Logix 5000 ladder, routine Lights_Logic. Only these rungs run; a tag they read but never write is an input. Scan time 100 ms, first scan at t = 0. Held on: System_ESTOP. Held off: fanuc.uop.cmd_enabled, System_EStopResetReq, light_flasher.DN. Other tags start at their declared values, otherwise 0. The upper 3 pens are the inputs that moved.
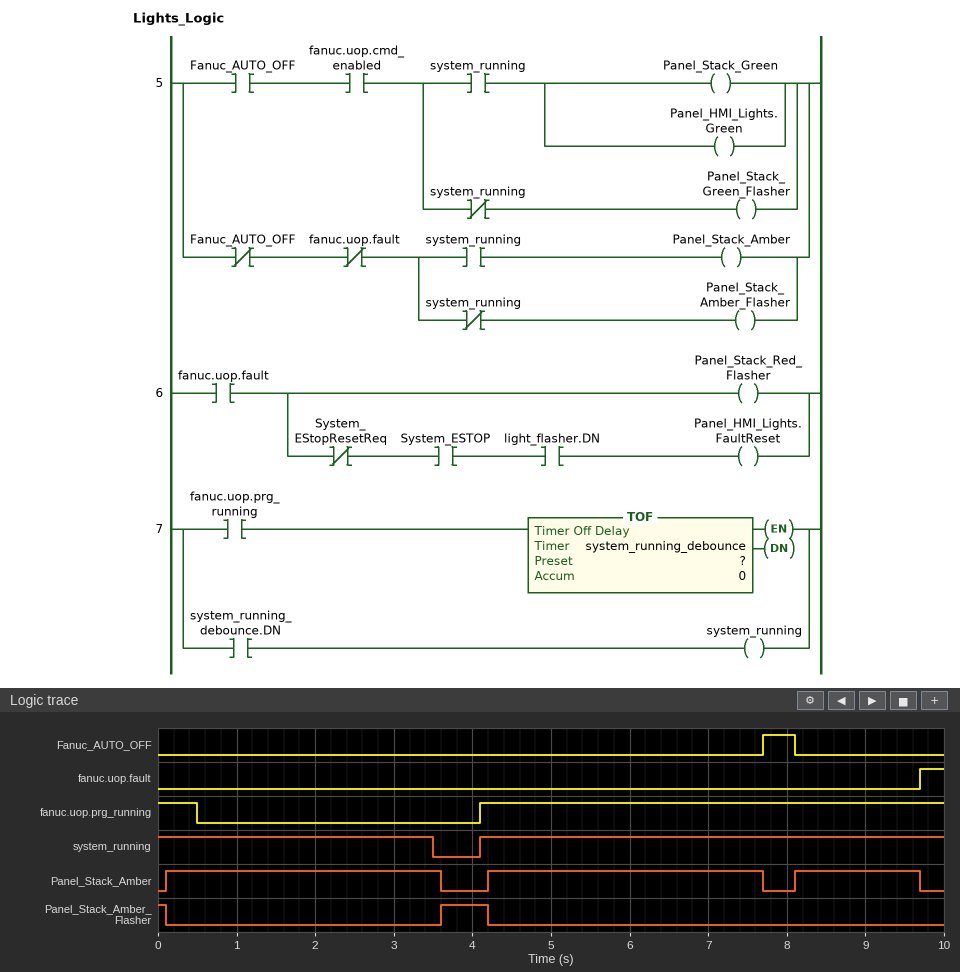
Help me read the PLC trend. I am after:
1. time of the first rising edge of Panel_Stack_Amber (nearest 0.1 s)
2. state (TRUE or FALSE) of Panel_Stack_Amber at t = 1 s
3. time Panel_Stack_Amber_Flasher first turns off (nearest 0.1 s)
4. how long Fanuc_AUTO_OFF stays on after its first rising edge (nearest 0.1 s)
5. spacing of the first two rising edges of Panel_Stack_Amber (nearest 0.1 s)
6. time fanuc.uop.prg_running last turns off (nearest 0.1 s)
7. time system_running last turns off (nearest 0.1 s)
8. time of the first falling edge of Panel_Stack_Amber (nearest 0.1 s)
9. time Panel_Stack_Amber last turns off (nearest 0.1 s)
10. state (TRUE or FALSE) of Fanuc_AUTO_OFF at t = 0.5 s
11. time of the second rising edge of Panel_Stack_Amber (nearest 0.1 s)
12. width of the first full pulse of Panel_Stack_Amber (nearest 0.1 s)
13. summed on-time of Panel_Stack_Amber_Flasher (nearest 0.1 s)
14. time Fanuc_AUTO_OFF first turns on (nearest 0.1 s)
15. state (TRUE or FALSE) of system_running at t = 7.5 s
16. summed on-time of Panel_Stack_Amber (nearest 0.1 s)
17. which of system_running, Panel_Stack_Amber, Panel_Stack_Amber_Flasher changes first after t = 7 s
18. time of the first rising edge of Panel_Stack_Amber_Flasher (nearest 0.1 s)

0.1 s
TRUE
0.1 s
0.4 s
4.1 s
0.5 s
3.5 s
3.6 s
9.7 s
FALSE
4.2 s
3.5 s
0.7 s
7.7 s
TRUE
8.6 s
Panel_Stack_Amber
3.6 s
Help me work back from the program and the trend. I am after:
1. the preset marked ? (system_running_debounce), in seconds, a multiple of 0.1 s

3.0 s
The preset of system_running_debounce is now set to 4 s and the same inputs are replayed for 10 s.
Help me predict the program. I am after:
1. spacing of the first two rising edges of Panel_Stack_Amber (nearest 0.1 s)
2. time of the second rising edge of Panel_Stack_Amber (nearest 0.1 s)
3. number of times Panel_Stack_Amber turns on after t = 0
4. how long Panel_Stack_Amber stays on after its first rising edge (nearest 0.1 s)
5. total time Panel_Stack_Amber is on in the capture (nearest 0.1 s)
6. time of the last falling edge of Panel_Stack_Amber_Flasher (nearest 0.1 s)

8.0 s
8.1 s
2
7.6 s
9.2 s
0.1 s
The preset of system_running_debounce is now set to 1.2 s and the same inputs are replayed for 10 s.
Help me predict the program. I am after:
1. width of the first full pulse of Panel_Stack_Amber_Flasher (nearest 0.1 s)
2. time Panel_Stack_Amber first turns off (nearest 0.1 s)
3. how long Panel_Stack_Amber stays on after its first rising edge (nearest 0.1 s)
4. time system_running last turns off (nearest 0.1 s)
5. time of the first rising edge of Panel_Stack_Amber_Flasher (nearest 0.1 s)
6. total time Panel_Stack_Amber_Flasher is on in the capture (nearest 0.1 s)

2.4 s
1.8 s
1.7 s
1.7 s
1.8 s
2.5 s
